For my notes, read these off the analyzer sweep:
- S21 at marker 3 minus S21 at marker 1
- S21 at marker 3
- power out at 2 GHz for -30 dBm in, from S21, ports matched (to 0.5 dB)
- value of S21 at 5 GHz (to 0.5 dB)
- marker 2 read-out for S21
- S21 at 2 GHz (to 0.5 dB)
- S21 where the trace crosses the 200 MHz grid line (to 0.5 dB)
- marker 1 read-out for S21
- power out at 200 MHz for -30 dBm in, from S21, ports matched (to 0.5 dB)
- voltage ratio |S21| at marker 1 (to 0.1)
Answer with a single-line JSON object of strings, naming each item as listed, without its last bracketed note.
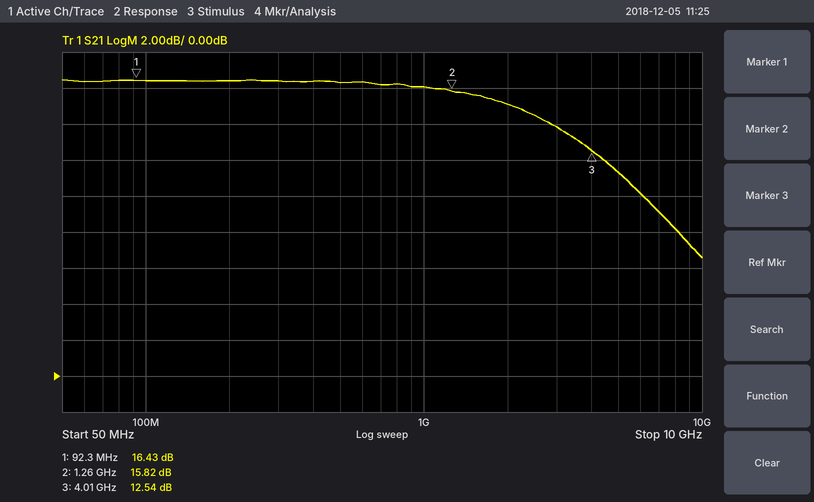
{"S21 at marker 3 minus S21 at marker 1": "-3.89 dB", "S21 at marker 3": "12.54 dB", "power out at 2 GHz for -30 dBm in, from S21, ports matched": "-15.0 dBm", "value of S21 at 5 GHz": "11.5 dB", "marker 2 read-out for S21": "15.82 dB", "S21 at 2 GHz": "15.0 dB", "S21 where the trace crosses the 200 MHz grid line": "16.5 dB", "marker 1 read-out for S21": "16.43 dB", "power out at 200 MHz for -30 dBm in, from S21, ports matched": "-13.5 dBm", "voltage ratio |S21| at marker 1": "6.6"}
